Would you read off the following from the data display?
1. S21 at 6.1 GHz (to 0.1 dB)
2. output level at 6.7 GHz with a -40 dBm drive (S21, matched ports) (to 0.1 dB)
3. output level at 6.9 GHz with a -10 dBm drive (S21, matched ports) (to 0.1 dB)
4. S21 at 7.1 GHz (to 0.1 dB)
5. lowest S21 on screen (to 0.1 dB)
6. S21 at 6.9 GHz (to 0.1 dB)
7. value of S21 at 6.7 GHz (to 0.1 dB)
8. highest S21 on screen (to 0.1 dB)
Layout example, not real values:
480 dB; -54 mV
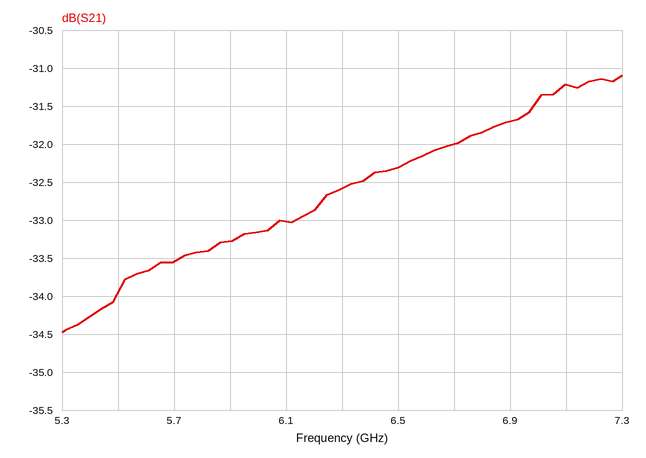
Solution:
-33.0 dB; -72.0 dBm; -41.7 dBm; -31.2 dB; -34.5 dB; -31.7 dB; -32.0 dB; -31.1 dB
